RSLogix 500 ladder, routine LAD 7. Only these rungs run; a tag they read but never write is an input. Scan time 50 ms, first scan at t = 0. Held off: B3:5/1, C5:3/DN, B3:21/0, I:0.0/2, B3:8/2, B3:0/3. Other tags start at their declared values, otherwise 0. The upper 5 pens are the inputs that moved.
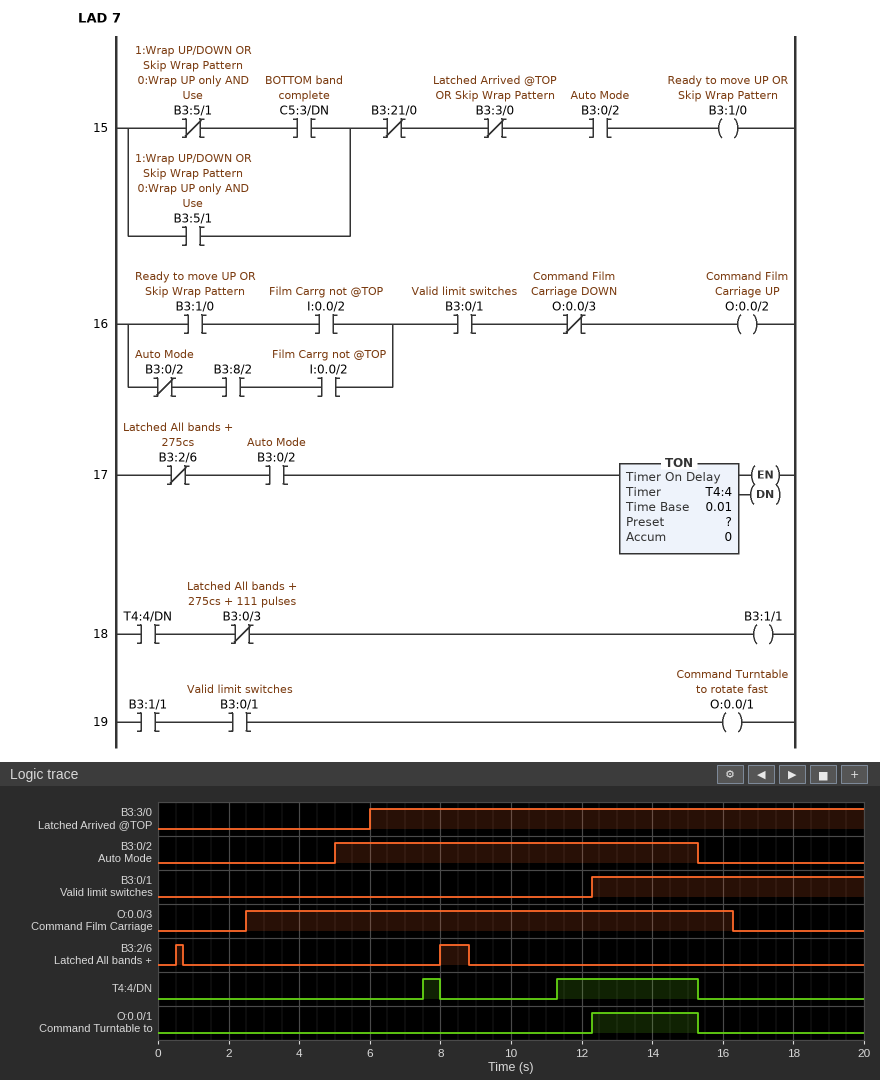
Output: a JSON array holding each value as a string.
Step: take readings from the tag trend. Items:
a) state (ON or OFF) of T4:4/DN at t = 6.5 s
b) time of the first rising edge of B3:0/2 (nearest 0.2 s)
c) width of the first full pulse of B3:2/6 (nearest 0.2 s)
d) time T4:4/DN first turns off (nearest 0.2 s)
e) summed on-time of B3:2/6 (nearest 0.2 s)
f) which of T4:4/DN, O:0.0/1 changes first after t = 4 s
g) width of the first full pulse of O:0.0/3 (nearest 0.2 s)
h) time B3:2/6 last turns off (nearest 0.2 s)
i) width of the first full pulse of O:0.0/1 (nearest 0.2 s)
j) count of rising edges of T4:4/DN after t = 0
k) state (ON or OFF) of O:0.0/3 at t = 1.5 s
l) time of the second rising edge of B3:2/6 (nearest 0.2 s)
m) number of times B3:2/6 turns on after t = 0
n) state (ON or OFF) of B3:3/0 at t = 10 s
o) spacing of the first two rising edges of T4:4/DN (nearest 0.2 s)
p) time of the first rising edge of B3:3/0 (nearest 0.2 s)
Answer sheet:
["OFF", "5.0 s", "0.2 s", "8.0 s", "1.0 s", "T4:4/DN", "13.8 s", "8.8 s", "3.0 s", "2", "OFF", "8.0 s", "2", "ON", "3.8 s", "6.0 s"]
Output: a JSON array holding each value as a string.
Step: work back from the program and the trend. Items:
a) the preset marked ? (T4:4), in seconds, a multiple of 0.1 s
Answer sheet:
["2.5 s"]
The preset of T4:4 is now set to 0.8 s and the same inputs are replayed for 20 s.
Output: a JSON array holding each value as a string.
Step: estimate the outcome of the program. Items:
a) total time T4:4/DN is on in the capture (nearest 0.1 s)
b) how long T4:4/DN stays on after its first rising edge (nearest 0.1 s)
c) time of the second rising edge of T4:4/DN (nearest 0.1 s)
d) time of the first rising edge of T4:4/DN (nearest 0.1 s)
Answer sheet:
["7.9 s", "2.2 s", "9.6 s", "5.8 s"]
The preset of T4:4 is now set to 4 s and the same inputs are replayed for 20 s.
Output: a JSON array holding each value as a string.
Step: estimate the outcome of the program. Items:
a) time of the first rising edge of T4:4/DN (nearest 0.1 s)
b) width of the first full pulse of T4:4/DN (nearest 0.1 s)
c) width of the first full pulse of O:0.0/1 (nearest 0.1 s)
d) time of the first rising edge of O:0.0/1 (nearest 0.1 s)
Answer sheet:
["12.8 s", "2.5 s", "2.5 s", "12.8 s"]
